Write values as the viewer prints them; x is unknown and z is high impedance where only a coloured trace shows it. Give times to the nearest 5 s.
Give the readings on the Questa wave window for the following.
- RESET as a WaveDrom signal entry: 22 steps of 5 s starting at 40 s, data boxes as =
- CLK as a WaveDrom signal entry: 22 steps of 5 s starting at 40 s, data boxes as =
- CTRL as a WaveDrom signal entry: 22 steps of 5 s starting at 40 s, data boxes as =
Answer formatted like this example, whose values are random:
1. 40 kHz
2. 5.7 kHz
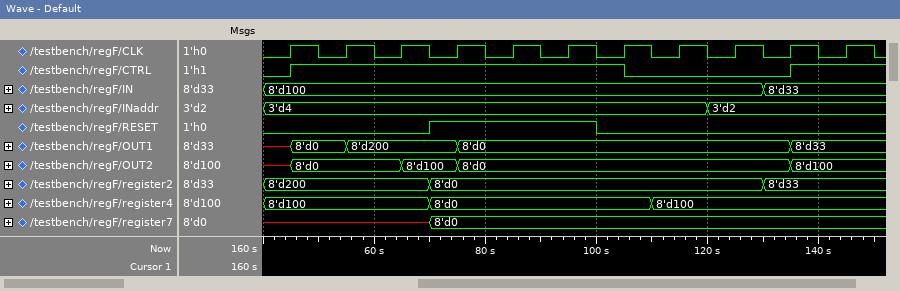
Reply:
1. {name: 'RESET', wave: '0.....1.....0.........'}
2. {name: 'CLK', wave: '0101010101010101010101'}
3. {name: 'CTRL', wave: '01...........0.....1..'}
